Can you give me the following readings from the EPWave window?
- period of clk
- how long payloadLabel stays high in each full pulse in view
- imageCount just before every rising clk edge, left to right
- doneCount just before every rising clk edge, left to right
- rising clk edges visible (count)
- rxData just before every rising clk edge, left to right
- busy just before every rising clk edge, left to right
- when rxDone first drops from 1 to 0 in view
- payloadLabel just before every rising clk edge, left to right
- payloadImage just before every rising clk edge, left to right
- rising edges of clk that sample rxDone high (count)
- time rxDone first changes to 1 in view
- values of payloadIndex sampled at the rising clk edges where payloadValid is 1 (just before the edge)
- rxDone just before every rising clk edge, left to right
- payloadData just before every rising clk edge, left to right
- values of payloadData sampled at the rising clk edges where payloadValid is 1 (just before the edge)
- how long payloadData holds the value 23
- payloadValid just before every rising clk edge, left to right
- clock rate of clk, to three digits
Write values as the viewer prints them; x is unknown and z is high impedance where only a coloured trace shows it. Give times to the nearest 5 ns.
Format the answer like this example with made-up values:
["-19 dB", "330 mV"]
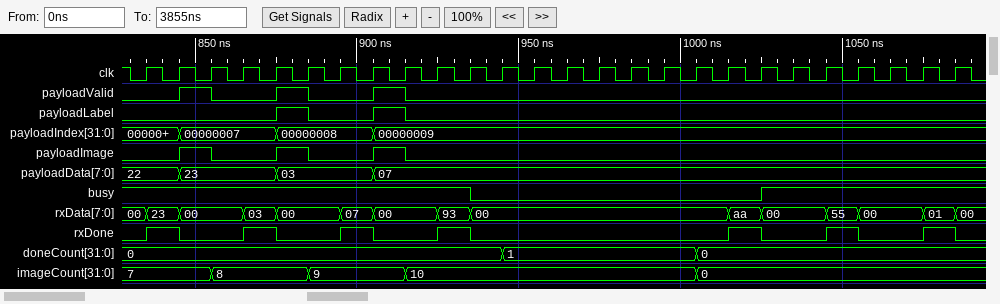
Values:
["10 ns", "10 ns, 10 ns", "7, 7, 7, 8, 8, 8, 9, 9, 9, 10, 10, 10, 10, 10, 10, 10, 10, 10, 0, 0, 0, 0, 0, 0, 0, 0", "0, 0, 0, 0, 0, 0, 0, 0, 0, 0, 0, 0, 1, 1, 1, 1, 1, 1, 0, 0, 0, 0, 0, 0, 0, 0", "26", "00, 23, 00, 00, 03, 00, 00, 07, 00, 00, 93, 00, 00, 00, 00, 00, 00, 00, 00, aa, 00, 00, 55, 00, 00, 01", "1 1 1 1 1 1 1 1 1 1 1 0 0 0 0 0 0 0 0 0 1 1 1 1 1 1", "845 ns", "0 0 0 0 0 1 0 0 1 0 0 0 0 0 0 0 0 0 0 0 0 0 0 0 0 0", "0 0 1 0 0 1 0 0 1 0 0 0 0 0 0 0 0 0 0 0 0 0 0 0 0 0", "7", "835 ns", "00000007, 00000008, 00000009", "0 1 0 0 1 0 0 1 0 0 1 0 0 0 0 0 0 0 0 1 0 0 1 0 0 1", "22, 22, 23, 23, 23, 03, 03, 03, 07, 07, 07, 07, 07, 07, 07, 07, 07, 07, 07, 07, 07, 07, 07, 07, 07, 07", "23, 03, 07", "30 ns", "0 0 1 0 0 1 0 0 1 0 0 0 0 0 0 0 0 0 0 0 0 0 0 0 0 0", "100 MHz"]
